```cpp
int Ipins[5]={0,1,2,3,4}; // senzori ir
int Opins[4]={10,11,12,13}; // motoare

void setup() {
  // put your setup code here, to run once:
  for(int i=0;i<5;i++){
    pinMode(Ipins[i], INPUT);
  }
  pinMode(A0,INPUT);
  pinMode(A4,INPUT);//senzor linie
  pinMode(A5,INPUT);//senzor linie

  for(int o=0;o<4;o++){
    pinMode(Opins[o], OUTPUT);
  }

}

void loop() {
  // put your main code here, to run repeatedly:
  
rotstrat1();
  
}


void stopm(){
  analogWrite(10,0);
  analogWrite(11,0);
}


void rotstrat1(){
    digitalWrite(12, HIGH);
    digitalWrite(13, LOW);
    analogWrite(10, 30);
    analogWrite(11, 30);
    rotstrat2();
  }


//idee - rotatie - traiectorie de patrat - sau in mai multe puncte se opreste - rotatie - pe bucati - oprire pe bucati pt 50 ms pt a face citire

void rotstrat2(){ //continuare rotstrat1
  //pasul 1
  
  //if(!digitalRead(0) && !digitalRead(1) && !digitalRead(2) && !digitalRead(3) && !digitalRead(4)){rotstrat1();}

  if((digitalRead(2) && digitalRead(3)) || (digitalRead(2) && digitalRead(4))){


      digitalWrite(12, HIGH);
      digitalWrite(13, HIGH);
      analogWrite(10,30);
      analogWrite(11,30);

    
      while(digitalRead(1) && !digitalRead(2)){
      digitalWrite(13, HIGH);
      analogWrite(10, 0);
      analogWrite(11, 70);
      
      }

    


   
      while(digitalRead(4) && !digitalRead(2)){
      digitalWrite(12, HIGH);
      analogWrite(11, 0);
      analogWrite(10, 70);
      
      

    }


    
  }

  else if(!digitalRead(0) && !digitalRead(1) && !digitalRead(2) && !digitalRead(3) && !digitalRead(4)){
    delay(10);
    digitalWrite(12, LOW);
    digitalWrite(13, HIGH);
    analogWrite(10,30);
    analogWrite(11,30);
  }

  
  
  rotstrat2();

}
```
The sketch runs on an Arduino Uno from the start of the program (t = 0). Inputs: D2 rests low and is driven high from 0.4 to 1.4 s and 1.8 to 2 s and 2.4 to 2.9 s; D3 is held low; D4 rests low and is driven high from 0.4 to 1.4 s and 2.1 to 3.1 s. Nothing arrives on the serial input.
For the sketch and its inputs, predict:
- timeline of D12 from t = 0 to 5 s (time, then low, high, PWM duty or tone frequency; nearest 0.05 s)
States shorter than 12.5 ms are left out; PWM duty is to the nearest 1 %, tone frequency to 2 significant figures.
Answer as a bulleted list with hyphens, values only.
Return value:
- 0 s low; 0.4 s high; 1.4 s low; 2.4 s high; 3.1 s low
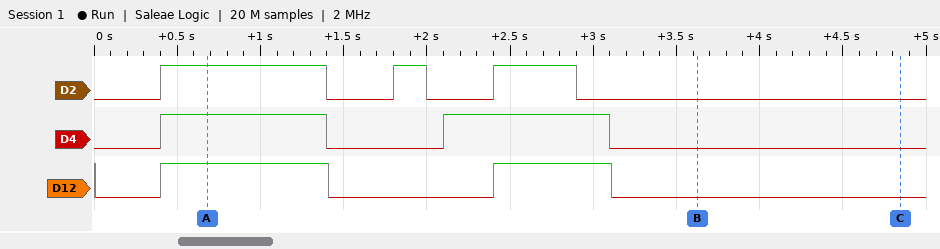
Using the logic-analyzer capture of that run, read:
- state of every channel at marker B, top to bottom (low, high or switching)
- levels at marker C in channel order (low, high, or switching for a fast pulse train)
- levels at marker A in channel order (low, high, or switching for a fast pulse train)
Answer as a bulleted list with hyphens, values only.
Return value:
- D2 low, D4 low, D12 low
- D2 low, D4 low, D12 low
- D2 high, D4 high, D12 high
